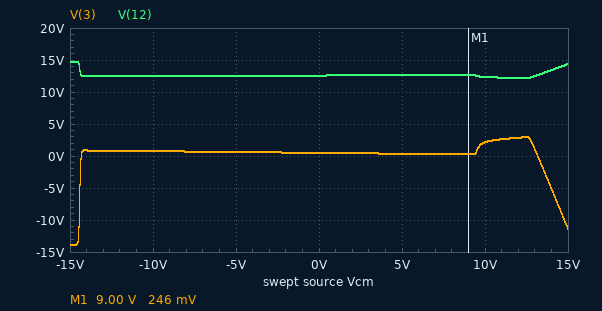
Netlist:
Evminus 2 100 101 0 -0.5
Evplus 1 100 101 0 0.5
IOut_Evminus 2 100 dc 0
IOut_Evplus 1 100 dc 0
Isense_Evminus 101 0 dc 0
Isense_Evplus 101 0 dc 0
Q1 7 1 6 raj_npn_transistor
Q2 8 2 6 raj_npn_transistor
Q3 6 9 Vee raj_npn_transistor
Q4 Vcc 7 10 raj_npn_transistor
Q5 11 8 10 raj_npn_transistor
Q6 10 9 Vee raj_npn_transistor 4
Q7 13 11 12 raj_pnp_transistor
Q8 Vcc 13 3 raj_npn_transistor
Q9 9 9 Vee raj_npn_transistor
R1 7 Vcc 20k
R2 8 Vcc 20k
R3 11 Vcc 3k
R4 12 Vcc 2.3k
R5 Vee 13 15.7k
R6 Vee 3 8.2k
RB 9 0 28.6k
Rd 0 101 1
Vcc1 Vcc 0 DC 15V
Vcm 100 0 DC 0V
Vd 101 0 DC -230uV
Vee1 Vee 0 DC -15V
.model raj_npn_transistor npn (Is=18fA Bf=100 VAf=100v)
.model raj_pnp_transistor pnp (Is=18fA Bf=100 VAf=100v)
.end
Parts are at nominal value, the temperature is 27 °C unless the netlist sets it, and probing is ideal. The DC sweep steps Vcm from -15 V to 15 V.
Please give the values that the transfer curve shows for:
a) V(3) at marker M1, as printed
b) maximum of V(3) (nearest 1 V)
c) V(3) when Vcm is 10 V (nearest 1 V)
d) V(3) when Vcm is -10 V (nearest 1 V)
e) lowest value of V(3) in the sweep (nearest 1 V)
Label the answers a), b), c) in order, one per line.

a) 246 mV
b) 3 V
c) 2 V
d) 1 V
e) -14 V
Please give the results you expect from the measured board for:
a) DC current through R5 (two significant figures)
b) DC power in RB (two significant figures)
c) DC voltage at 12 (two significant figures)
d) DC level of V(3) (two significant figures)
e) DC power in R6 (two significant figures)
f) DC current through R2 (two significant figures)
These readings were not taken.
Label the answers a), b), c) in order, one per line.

a) 1.0 mA
b) 7.2 mW
c) 13 V
d) 490 mV
e) 29 mW
f) 280 µA
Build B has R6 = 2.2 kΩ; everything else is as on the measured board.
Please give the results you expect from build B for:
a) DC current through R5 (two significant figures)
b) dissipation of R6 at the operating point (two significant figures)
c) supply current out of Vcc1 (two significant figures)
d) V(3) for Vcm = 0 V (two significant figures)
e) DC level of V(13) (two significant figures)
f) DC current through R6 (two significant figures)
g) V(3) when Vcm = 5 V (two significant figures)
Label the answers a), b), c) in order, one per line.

a) 990 µA
b) 100 mW
c) 11 mA
d) -200 mV
e) 490 mV
f) 6.7 mA
g) -330 mV
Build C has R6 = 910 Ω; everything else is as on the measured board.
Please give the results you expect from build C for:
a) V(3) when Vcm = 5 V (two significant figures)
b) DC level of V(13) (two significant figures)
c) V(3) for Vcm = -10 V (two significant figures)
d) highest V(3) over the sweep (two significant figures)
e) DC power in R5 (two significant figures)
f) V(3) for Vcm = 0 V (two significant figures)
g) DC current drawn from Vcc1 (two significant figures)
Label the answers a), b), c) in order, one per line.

a) -1.4 V
b) -620 mV
c) -1.1 V
d) 840 mV
e) 13 mW
f) -1.3 V
g) 19 mA
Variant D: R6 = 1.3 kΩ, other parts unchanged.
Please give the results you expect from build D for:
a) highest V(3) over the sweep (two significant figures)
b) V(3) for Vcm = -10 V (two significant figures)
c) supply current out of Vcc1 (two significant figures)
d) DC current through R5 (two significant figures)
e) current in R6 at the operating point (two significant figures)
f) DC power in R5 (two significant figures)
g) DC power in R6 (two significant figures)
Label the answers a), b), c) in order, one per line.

a) 1.5 V
b) -530 mV
c) 15 mA
d) 950 µA
e) 11 mA
f) 14 mW
g) 160 mW
